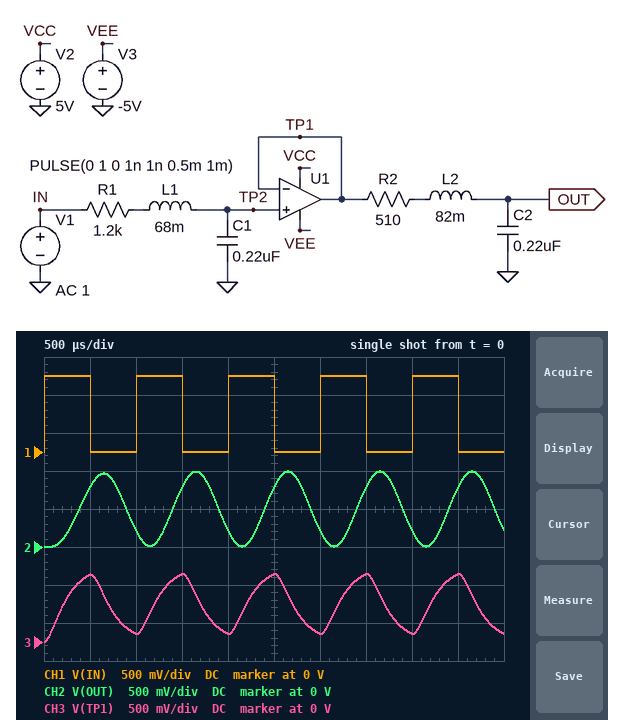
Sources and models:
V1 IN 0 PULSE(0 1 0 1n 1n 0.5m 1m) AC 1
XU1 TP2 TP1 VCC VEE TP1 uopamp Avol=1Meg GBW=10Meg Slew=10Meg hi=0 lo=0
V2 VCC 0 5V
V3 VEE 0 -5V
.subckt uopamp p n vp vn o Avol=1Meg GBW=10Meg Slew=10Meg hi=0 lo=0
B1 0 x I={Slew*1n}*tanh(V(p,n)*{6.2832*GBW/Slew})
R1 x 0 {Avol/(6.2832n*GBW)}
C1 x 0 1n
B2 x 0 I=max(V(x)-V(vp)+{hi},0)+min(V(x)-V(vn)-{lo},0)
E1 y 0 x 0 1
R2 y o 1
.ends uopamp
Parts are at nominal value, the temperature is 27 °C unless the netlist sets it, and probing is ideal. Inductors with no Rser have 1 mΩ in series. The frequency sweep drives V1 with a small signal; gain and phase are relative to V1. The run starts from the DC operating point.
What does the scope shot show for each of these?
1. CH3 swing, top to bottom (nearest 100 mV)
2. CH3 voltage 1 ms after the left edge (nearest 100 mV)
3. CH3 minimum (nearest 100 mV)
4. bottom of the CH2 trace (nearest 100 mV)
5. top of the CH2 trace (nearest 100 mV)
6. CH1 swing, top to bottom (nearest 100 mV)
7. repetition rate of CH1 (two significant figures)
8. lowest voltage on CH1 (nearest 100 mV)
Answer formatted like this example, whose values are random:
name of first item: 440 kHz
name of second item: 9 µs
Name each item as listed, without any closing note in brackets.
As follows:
CH3 swing, top to bottom: 900 mV
CH3 voltage 1 ms after the left edge: 100 mV
CH3 minimum: 0 V
bottom of the CH2 trace: 0 V
top of the CH2 trace: 1.0 V
CH1 swing, top to bottom: 1.0 V
repetition rate of CH1: 1.0 kHz
lowest voltage on CH1: 0 V
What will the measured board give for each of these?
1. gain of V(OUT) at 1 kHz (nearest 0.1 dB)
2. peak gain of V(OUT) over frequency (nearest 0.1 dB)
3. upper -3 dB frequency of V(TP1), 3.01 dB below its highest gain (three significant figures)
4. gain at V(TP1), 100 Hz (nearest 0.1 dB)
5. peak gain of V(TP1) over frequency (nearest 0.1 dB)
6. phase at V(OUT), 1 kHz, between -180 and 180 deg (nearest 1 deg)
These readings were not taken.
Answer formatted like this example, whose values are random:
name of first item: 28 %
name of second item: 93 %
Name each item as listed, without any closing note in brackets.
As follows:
gain of V(OUT) at 1 kHz: -2.3 dB
peak gain of V(OUT) over frequency: 0 dB
upper -3 dB frequency of V(TP1), 3.01 dB below its highest gain: 752 Hz
gain at V(TP1), 100 Hz: -0.1 dB
peak gain of V(TP1) over frequency: 0 dB
phase at V(OUT), 1 kHz, between -180 and 180 deg: -144 deg
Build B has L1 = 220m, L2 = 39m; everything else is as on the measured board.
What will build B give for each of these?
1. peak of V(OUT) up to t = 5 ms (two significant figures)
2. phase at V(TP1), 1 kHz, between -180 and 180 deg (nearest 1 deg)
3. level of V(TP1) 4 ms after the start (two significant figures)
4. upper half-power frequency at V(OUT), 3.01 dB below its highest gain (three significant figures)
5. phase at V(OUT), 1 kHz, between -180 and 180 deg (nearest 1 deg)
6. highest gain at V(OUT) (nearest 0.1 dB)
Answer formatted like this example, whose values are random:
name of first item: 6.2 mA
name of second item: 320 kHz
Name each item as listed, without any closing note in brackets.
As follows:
peak of V(OUT) up to t = 5 ms: 920 mV
phase at V(TP1), 1 kHz, between -180 and 180 deg: -119 deg
level of V(TP1) 4 ms after the start: 200 mV
upper half-power frequency at V(OUT), 3.01 dB below its highest gain: 820 Hz
phase at V(OUT), 1 kHz, between -180 and 180 deg: -166 deg
highest gain at V(OUT): 0.5 dB
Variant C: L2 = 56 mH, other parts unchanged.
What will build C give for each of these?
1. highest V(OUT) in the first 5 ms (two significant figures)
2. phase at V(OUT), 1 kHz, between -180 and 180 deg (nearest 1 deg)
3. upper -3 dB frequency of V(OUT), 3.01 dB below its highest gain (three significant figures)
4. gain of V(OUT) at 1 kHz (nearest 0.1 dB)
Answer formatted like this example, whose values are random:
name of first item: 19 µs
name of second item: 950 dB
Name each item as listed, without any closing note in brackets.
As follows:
highest V(OUT) in the first 5 ms: 930 mV
phase at V(OUT), 1 kHz, between -180 and 180 deg: -130 deg
upper -3 dB frequency of V(OUT), 3.01 dB below its highest gain: 928 Hz
gain of V(OUT) at 1 kHz: -3.5 dB
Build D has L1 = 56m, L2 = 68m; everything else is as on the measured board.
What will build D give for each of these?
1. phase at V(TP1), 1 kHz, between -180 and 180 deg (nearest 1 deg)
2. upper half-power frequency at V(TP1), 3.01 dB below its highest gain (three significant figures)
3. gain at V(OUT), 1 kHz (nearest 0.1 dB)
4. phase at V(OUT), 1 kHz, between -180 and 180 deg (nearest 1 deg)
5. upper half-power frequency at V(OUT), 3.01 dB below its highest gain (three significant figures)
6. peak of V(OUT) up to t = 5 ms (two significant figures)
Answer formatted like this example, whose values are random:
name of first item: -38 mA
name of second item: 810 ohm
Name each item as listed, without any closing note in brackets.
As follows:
phase at V(TP1), 1 kHz, between -180 and 180 deg: -73 deg
upper half-power frequency at V(TP1), 3.01 dB below its highest gain: 725 Hz
gain at V(OUT), 1 kHz: -3.0 dB
phase at V(OUT), 1 kHz, between -180 and 180 deg: -133 deg
upper half-power frequency at V(OUT), 3.01 dB below its highest gain: 999 Hz
peak of V(OUT) up to t = 5 ms: 950 mV
